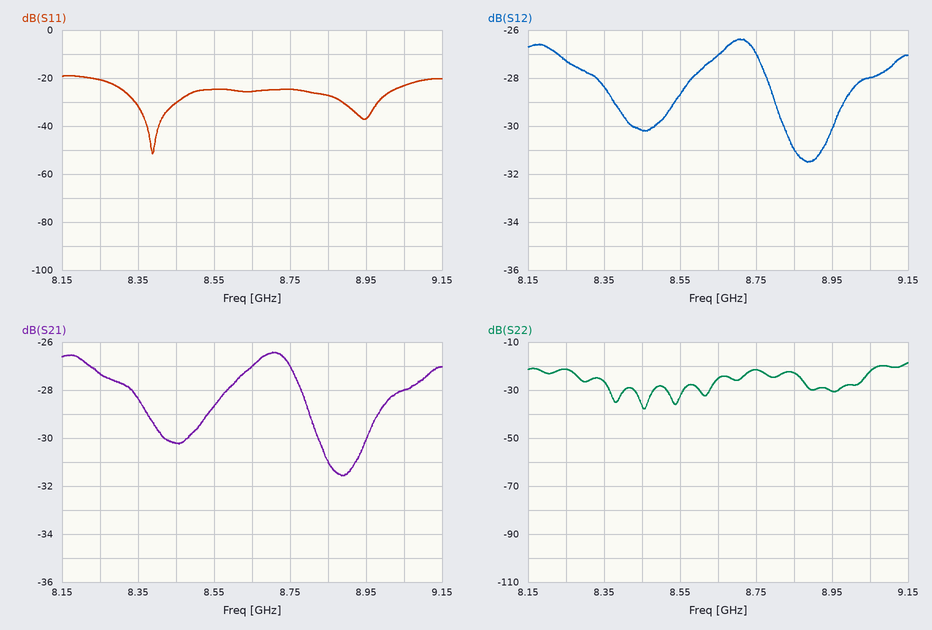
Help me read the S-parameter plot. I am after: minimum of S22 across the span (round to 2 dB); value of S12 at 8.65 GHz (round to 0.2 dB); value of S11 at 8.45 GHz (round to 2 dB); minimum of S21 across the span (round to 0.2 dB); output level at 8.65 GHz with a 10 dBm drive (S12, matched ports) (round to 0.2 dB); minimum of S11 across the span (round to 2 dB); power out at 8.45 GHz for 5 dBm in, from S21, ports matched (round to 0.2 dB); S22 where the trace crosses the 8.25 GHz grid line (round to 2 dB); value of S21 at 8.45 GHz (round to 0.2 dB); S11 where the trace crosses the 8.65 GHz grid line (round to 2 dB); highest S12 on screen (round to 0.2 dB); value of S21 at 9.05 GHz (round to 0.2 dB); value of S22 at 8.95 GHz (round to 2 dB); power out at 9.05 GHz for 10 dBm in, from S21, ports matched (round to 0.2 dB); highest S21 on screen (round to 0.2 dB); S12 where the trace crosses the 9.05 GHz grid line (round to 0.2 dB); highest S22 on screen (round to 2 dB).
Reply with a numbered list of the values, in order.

1. -38 dB
2. -27.0 dB
3. -30 dB
4. -31.6 dB
5. -17.0 dBm
6. -52 dB
7. -25.2 dBm
8. -22 dB
9. -30.2 dB
10. -26 dB
11. -26.4 dB
12. -28.0 dB
13. -30 dB
14. -18.0 dBm
15. -26.4 dB
16. -28.0 dB
17. -18 dB
